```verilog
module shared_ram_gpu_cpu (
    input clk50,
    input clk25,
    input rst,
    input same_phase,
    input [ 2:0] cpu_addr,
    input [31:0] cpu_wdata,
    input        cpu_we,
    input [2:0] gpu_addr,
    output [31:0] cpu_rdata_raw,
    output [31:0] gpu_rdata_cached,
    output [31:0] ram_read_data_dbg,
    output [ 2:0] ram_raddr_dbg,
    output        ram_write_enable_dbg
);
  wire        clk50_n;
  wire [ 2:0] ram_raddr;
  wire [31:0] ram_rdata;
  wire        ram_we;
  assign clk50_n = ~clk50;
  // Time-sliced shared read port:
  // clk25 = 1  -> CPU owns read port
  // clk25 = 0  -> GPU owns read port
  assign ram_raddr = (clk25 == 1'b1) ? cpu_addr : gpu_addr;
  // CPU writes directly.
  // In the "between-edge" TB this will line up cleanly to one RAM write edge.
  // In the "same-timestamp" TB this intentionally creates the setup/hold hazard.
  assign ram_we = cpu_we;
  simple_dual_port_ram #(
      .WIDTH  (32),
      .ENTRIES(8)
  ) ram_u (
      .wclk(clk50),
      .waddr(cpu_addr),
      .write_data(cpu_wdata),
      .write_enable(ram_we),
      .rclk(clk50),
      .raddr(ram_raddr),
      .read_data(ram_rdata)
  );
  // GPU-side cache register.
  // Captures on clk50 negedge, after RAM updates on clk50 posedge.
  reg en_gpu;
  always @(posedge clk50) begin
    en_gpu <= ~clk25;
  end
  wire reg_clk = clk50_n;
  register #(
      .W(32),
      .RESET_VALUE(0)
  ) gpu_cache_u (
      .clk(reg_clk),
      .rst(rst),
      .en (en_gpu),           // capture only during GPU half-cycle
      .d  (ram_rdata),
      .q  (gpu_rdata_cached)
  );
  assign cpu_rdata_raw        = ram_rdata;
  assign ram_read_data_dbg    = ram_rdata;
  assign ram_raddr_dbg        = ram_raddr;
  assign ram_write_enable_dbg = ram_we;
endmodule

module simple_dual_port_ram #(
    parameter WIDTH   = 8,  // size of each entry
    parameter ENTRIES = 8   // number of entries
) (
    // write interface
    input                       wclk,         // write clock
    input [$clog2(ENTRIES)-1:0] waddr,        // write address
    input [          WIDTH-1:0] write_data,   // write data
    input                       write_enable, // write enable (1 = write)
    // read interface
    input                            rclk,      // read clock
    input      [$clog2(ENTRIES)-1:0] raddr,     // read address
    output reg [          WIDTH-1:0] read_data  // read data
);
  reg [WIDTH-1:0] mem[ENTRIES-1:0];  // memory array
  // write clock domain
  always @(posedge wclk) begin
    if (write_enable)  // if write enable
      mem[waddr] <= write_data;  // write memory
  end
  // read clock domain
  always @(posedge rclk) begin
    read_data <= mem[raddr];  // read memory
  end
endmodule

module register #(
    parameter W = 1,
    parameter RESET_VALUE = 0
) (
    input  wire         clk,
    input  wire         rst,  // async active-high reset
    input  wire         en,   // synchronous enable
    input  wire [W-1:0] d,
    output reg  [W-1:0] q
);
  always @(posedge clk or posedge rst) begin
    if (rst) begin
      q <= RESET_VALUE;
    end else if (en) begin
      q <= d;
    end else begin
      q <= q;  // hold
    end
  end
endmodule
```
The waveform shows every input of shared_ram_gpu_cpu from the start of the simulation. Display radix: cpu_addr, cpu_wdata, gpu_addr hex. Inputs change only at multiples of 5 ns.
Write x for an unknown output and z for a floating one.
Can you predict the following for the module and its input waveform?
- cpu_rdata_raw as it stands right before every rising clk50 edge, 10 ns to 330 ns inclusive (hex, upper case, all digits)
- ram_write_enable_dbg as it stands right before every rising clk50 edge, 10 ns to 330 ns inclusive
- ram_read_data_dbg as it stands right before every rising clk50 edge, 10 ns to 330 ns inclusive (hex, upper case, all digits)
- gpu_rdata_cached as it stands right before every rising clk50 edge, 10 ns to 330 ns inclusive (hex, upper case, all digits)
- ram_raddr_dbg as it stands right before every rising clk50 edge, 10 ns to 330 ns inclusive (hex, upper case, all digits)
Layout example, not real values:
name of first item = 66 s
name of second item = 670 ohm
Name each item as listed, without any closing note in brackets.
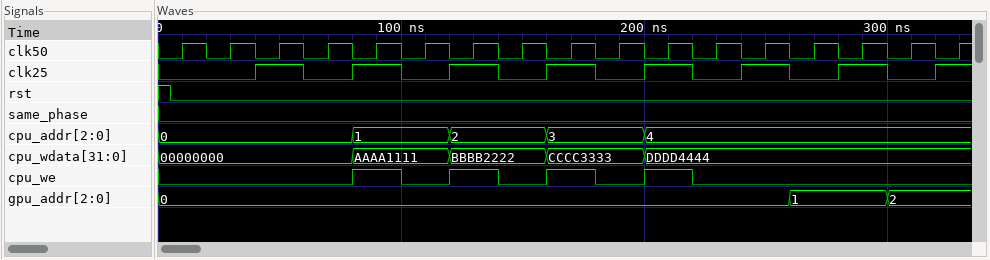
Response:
cpu_rdata_raw as it stands right before every rising clk50 edge, 10 ns to 330 ns inclusive = x, x, x, x, x, x, x, x, x, x, x, x, x, DDDD4444, AAAA1111, DDDD4444, BBBB2222
ram_write_enable_dbg as it stands right before every rising clk50 edge, 10 ns to 330 ns inclusive = 0 0 0 0 1 0 1 0 1 0 1 0 0 0 0 0 0
ram_read_data_dbg as it stands right before every rising clk50 edge, 10 ns to 330 ns inclusive = x, x, x, x, x, x, x, x, x, x, x, x, x, DDDD4444, AAAA1111, DDDD4444, BBBB2222
gpu_rdata_cached as it stands right before every rising clk50 edge, 10 ns to 330 ns inclusive = 00000000, x, x, x, x, x, x, x, x, x, x, x, x, x, AAAA1111, AAAA1111, BBBB2222
ram_raddr_dbg as it stands right before every rising clk50 edge, 10 ns to 330 ns inclusive = 0, 0, 0, 0, 1, 0, 2, 0, 3, 0, 4, 0, 4, 1, 4, 2, 4
